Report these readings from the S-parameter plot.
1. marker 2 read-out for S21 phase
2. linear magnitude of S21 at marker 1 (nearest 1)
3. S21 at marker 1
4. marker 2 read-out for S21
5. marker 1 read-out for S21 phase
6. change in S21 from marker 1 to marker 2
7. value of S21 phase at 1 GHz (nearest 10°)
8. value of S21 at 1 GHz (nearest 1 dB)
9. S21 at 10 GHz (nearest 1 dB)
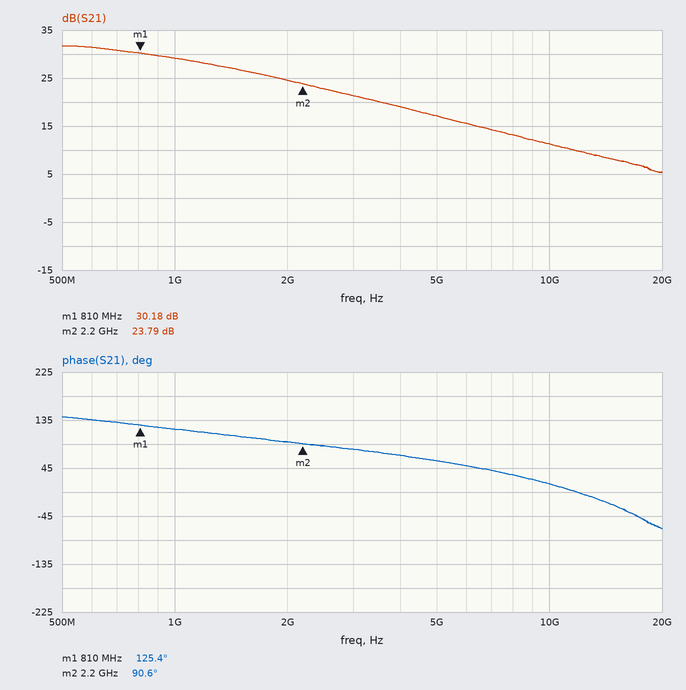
90.6°
32
30.18 dB
23.79 dB
125.4°
-6.39 dB
120°
29 dB
11 dB
